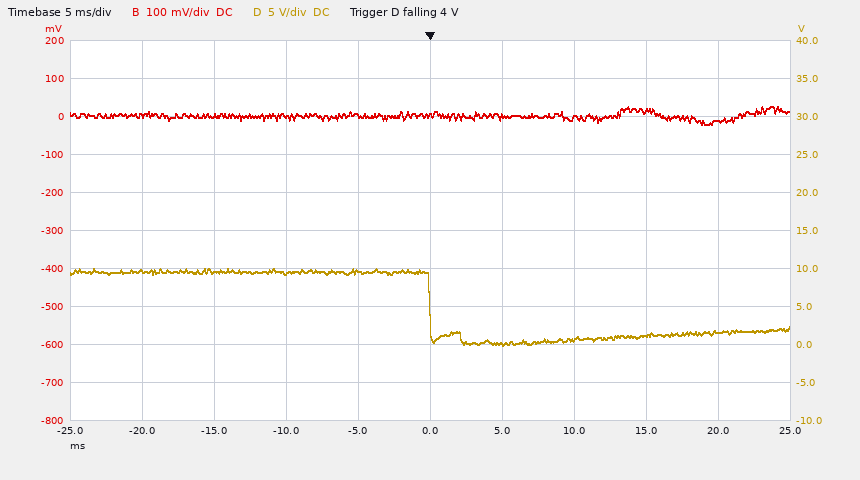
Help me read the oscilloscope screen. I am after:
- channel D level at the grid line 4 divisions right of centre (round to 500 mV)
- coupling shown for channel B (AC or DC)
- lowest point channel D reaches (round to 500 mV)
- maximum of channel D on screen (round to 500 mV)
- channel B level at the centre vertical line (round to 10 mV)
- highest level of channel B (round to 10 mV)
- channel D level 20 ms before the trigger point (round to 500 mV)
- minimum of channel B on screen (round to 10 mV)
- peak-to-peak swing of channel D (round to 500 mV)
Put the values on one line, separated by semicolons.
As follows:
1.5 V; DC; 0.0 V; 10.0 V; 0 mV; 30 mV; 9.5 V; -20 mV; 10.0 V
